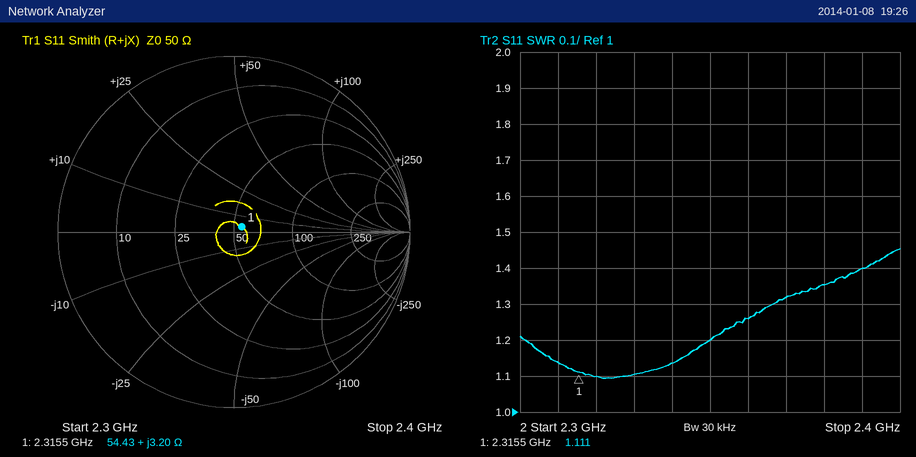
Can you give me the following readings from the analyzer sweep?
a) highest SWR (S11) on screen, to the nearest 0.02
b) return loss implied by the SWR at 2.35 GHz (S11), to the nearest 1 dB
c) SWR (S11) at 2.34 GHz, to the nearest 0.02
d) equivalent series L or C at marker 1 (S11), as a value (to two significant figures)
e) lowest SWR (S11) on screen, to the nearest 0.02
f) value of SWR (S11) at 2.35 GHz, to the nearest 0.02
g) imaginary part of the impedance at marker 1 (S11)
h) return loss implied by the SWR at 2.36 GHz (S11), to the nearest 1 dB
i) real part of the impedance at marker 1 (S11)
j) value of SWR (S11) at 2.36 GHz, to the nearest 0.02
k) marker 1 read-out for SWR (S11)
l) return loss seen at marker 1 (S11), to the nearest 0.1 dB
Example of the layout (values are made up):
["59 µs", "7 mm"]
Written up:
["1.46", "21 dB", "1.14", "220 pH", "1.10", "1.20", "+3.20 Ω", "19 dB", "54.43 Ω", "1.26", "1.111", "25.6 dB"]
